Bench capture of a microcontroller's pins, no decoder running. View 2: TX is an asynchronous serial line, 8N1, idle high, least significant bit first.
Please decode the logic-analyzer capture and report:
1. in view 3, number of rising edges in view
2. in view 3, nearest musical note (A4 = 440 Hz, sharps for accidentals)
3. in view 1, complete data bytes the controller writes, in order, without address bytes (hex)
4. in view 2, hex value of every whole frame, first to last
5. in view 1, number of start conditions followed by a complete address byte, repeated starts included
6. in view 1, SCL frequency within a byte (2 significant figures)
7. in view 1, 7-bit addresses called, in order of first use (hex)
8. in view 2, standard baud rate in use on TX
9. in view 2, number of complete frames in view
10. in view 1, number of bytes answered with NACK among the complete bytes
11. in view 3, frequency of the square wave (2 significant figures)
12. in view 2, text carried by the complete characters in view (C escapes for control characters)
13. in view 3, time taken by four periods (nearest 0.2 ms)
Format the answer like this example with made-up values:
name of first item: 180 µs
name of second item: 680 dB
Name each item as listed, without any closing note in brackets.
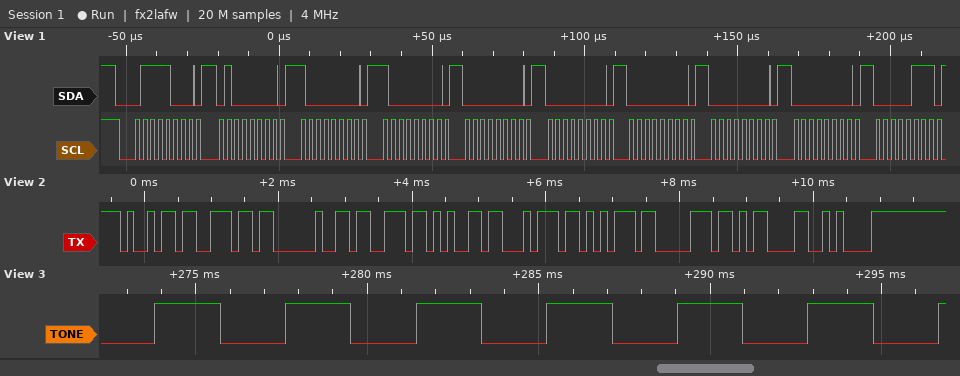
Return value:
in view 3, number of rising edges in view: 7
in view 3, nearest musical note: C4
in view 1, complete data bytes the controller writes, in order, without address bytes: 40 80 80 00 00 00 00 00 07
in view 2, hex value of every whole frame, first to last: 69 6E 20 73 65 74 75 70 0D 0A
in view 1, number of start conditions followed by a complete address byte, repeated starts included: 1
in view 1, SCL frequency within a byte: 400 kHz
in view 1, 7-bit addresses called, in order of first use: 0x3C
in view 2, standard baud rate in use on TX: 9600 baud
in view 2, number of complete frames in view: 10
in view 1, number of bytes answered with NACK among the complete bytes: 0
in view 3, frequency of the square wave: 260 Hz
in view 2, text carried by the complete characters in view: "in setup\r\n"
in view 3, time taken by four periods: 15.2 ms
